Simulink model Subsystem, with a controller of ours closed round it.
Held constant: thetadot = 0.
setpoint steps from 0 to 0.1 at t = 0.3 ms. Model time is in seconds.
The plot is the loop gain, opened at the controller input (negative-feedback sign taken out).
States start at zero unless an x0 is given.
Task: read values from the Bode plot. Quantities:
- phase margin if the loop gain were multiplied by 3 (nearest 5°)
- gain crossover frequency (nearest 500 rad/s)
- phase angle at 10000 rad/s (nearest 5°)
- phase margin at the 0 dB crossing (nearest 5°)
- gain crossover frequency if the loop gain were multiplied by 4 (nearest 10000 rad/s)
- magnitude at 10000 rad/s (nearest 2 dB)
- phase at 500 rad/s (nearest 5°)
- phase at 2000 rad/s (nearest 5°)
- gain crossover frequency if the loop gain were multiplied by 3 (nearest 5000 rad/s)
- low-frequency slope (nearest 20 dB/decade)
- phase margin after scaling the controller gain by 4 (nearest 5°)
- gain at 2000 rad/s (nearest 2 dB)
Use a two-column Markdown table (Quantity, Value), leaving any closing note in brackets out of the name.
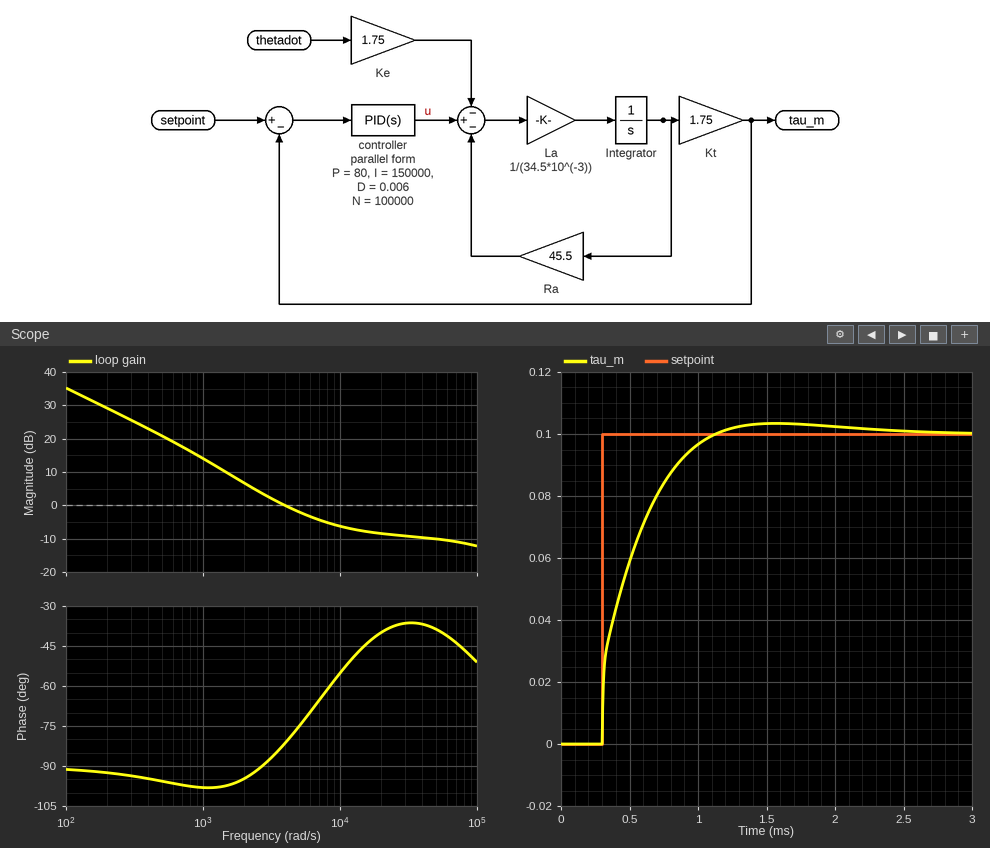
| Quantity | Value |
|---|---|
| phase margin if the loop gain were multiplied by 3 | 145° |
| gain crossover frequency | 4000 rad/s |
| phase angle at 10000 rad/s | -55° |
| phase margin at the 0 dB crossing | 100° |
| gain crossover frequency if the loop gain were multiplied by 4 | 100000 rad/s |
| magnitude at 10000 rad/s | -6 dB |
| phase at 500 rad/s | -95° |
| phase at 2000 rad/s | -95° |
| gain crossover frequency if the loop gain were multiplied by 3 | 40000 rad/s |
| low-frequency slope | -20 dB/decade |
| phase margin after scaling the controller gain by 4 | 130° |
| gain at 2000 rad/s | 6 dB |
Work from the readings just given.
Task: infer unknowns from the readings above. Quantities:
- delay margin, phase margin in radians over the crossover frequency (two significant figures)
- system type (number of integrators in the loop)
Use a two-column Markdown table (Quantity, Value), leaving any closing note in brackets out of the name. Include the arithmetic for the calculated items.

| Quantity | Value |
|---|---|
| delay margin, phase margin in radians over the crossover frequency | 100 × π / 180 / 4000 = 0.00044 s |
| system type | 1 |
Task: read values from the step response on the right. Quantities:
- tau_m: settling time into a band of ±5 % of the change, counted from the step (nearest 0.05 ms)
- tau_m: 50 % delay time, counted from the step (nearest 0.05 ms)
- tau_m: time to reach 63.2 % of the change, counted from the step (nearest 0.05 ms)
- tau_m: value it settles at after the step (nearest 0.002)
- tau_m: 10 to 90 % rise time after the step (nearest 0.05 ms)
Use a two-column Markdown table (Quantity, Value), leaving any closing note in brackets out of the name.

| Quantity | Value |
|---|---|
| tau_m: settling time into a band of ±5 % of the change, counted from the step | 0.65 ms |
| tau_m: 50 % delay time, counted from the step | 0.15 ms |
| tau_m: time to reach 63.2 % of the change, counted from the step | 0.25 ms |
| tau_m: value it settles at after the step | 0.100 |
| tau_m: 10 to 90 % rise time after the step | 0.55 ms |
